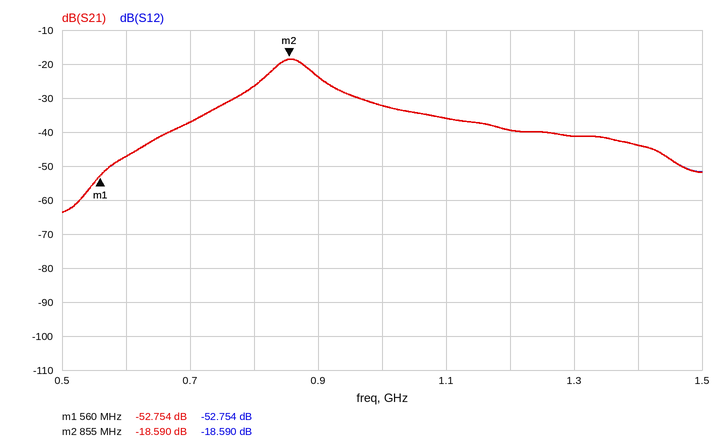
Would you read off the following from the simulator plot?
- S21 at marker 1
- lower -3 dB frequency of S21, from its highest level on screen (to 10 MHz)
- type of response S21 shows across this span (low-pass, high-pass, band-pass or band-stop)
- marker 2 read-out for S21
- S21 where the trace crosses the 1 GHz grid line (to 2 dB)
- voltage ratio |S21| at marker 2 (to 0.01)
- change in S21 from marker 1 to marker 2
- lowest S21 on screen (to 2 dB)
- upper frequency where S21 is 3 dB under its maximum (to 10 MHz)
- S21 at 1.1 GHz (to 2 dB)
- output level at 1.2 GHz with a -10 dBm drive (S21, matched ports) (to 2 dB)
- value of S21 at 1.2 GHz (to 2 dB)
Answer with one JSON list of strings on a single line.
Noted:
["-52.754 dB", "830 MHz", "band-pass", "-18.590 dB", "-32 dB", "0.12", "34.164 dB", "-64 dB", "890 MHz", "-36 dB", "-50 dBm", "-40 dB"]
